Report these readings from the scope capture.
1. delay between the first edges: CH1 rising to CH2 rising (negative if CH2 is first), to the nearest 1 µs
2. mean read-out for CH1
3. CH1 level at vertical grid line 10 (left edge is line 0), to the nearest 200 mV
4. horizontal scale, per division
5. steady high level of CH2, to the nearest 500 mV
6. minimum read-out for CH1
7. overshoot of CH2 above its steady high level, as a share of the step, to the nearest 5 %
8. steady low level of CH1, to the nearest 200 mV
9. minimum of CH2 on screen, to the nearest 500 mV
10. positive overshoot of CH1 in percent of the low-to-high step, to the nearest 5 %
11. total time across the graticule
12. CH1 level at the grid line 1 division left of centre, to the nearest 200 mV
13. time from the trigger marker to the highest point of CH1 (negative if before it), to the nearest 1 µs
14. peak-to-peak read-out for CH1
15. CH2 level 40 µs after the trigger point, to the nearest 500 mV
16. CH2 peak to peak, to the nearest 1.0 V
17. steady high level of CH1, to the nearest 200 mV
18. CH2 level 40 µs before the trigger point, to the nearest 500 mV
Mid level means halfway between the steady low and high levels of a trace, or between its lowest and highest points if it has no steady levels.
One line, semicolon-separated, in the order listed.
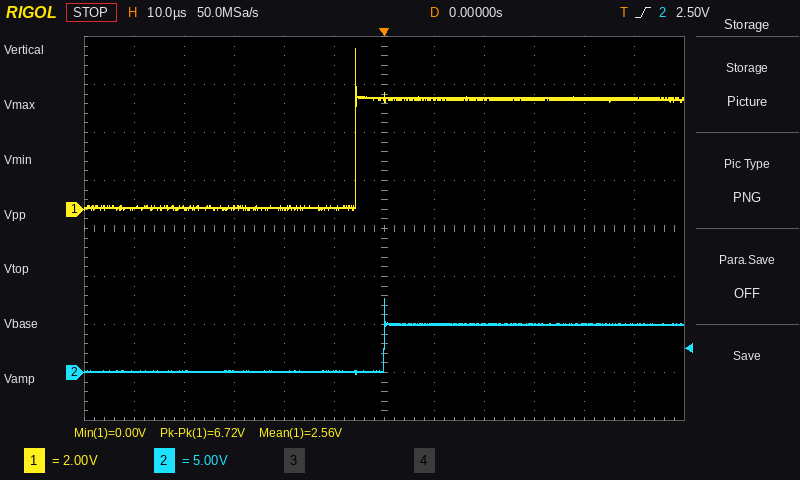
+6 µs; 2.56 V; 4.6 V; 10 µs; 5.0 V; 0.00 V; 55 %; 0.0 V; 0.0 V; 45 %; 120 µs; 0.0 V; -6 µs; 6.72 V; 5.0 V; 8.0 V; 4.6 V; 0.0 V
